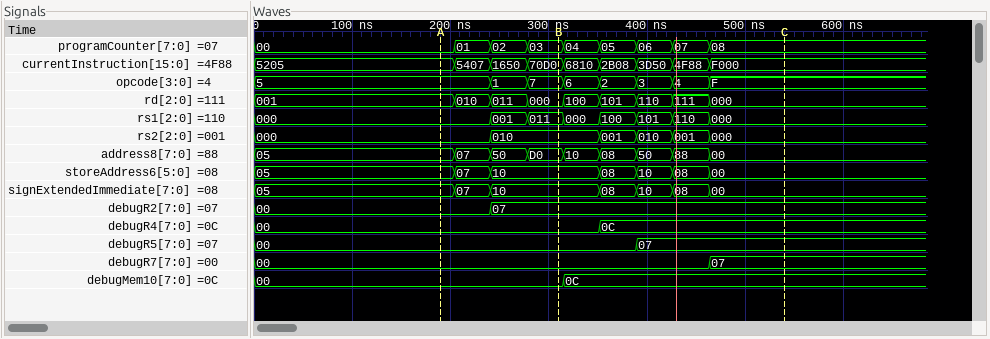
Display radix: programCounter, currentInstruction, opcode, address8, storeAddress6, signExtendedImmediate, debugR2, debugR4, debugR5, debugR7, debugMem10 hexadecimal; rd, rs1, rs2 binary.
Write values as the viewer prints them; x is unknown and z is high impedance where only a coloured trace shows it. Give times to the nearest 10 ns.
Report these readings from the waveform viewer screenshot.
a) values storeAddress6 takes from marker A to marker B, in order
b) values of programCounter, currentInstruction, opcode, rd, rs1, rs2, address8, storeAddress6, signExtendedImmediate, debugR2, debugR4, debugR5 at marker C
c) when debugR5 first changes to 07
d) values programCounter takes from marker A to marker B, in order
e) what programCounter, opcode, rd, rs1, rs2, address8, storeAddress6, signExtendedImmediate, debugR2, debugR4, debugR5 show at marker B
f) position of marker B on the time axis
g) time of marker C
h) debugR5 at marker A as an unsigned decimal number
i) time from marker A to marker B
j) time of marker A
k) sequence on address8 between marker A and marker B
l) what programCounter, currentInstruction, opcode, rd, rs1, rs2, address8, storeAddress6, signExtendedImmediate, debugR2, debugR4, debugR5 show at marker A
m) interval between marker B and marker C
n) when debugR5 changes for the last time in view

05, 07, 10
programCounter=08, currentInstruction=F000, opcode=F, rd=000, rs1=000, rs2=000, address8=00, storeAddress6=00, signExtendedImmediate=00, debugR2=07, debugR4=0C, debugR5=07
390 ns
00, 01, 02, 03
programCounter=03, opcode=7, rd=000, rs1=011, rs2=010, address8=D0, storeAddress6=10, signExtendedImmediate=10, debugR2=07, debugR4=00, debugR5=00
310 ns
540 ns
0
120 ns
190 ns
05, 07, 50, D0
programCounter=00, currentInstruction=5205, opcode=5, rd=001, rs1=000, rs2=000, address8=05, storeAddress6=05, signExtendedImmediate=05, debugR2=00, debugR4=00, debugR5=00
230 ns
390 ns
